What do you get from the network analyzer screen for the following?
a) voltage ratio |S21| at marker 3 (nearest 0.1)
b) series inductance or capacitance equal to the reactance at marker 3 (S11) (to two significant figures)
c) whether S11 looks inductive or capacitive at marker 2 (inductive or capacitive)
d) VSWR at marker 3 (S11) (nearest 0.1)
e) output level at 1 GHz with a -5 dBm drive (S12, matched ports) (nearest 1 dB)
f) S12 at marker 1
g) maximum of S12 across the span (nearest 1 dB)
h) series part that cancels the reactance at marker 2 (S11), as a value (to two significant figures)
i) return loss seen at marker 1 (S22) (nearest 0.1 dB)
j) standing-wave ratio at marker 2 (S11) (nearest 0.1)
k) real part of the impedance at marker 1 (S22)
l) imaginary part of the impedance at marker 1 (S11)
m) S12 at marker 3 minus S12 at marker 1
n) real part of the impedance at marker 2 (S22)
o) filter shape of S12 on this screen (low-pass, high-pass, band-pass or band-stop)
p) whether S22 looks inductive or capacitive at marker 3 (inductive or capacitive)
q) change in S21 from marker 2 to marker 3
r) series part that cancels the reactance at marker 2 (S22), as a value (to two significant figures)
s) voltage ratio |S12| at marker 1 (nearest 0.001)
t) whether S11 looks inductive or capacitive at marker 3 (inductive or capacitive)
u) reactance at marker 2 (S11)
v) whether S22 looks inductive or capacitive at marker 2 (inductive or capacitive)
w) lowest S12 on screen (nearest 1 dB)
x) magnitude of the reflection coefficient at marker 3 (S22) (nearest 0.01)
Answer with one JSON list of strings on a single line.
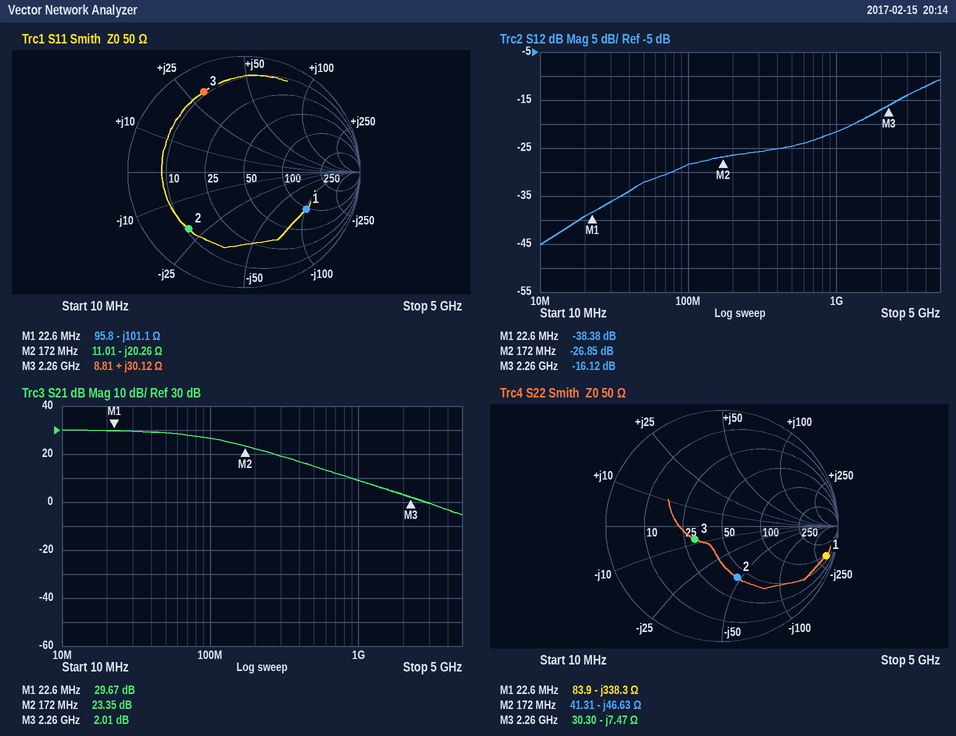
["1.3", "2.1 nH", "capacitive", "7.8", "-27 dBm", "-38.38 dB", "-11 dB", "19 nH", "0.6 dB", "5.3", "83.9 Ω", "-101.1 Ω", "22.26 dB", "41.31 Ω", "high-pass", "capacitive", "-21.34 dB", "43 nH", "0.012", "inductive", "-20.26 Ω", "capacitive", "-45 dB", "0.26"]
